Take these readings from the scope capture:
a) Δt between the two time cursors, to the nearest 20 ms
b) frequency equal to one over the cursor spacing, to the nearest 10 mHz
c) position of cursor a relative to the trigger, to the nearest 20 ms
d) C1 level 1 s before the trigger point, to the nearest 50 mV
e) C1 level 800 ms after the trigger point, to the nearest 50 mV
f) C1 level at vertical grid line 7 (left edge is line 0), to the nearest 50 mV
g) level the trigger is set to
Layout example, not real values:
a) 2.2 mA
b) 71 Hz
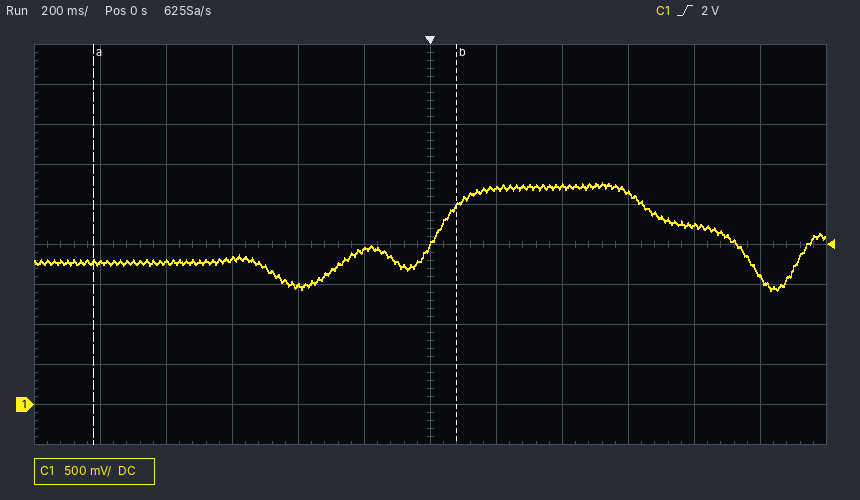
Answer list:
a) 1.10 s
b) 910 mHz
c) -1.02 s
d) 1.75 V
e) 2.25 V
f) 2.70 V
g) 2 V
